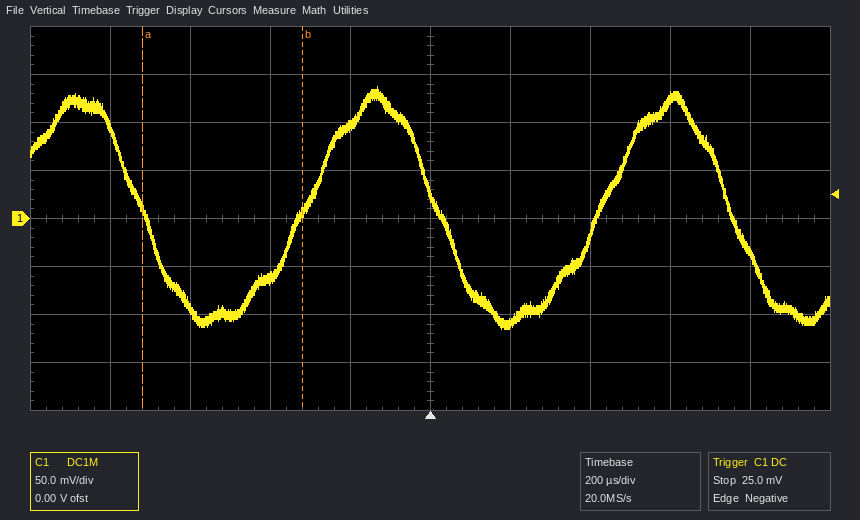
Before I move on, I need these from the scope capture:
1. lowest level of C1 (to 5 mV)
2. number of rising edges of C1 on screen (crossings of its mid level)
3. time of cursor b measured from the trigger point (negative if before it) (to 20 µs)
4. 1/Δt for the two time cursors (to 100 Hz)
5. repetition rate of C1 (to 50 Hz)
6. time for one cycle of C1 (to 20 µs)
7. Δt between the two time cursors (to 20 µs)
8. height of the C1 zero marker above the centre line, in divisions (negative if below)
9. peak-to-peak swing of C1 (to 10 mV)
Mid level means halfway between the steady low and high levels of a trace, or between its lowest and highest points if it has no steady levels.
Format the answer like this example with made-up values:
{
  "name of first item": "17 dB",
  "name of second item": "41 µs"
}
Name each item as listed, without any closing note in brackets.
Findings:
{
  "lowest level of C1": "-115 mV",
  "number of rising edges of C1 on screen": "2",
  "time of cursor b measured from the trigger point (negative if before it)": "-320 µs",
  "1/Δt for the two time cursors": "2.5 kHz",
  "repetition rate of C1": "1.35 kHz",
  "time for one cycle of C1": "740 µs",
  "Δt between the two time cursors": "400 µs",
  "height of the C1 zero marker above the centre line, in divisions": "0.0 div",
  "peak-to-peak swing of C1": "250 mV"
}
